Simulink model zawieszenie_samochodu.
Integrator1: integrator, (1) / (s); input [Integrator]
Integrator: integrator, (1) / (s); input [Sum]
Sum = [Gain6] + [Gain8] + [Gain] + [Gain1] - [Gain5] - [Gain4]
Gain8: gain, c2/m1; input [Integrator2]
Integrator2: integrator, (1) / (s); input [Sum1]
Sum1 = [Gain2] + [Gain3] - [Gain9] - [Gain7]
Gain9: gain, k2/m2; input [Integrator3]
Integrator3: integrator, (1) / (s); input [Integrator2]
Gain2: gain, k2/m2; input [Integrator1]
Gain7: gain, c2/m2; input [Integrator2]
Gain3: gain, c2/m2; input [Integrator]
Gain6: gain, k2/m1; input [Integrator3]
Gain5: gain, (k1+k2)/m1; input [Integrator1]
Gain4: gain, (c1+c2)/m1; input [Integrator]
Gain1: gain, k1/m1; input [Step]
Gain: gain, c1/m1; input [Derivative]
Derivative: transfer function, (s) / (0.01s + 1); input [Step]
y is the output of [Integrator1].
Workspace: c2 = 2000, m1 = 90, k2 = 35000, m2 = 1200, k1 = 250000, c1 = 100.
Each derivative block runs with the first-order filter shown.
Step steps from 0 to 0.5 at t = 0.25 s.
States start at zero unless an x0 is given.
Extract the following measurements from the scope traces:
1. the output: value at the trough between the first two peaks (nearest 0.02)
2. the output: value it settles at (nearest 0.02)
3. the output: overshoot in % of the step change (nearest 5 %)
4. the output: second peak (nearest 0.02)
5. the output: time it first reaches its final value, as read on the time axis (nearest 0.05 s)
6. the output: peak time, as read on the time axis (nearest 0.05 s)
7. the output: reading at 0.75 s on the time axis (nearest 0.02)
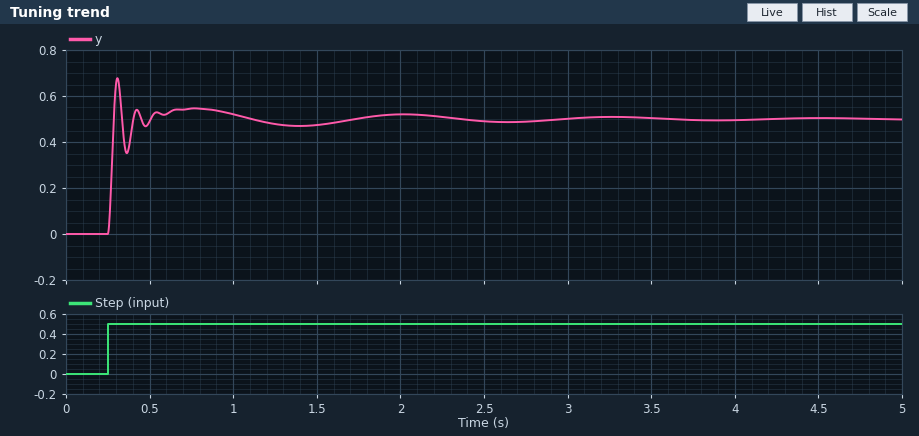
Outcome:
0.36
0.50
35 %
0.54
0.30 s
0.30 s
0.54
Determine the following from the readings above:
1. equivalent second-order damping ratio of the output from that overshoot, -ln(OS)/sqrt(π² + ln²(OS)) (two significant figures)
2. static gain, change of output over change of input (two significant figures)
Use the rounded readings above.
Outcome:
0.32
1.0
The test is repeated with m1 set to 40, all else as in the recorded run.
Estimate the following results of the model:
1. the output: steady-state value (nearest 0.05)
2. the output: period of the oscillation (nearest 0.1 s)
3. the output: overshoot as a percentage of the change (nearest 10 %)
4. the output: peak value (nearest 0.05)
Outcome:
0.50
0.5 s
20 %
0.60
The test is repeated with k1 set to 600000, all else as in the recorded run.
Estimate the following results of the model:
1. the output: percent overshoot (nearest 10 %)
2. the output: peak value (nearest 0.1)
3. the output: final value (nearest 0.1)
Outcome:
60 %
0.8
0.5
